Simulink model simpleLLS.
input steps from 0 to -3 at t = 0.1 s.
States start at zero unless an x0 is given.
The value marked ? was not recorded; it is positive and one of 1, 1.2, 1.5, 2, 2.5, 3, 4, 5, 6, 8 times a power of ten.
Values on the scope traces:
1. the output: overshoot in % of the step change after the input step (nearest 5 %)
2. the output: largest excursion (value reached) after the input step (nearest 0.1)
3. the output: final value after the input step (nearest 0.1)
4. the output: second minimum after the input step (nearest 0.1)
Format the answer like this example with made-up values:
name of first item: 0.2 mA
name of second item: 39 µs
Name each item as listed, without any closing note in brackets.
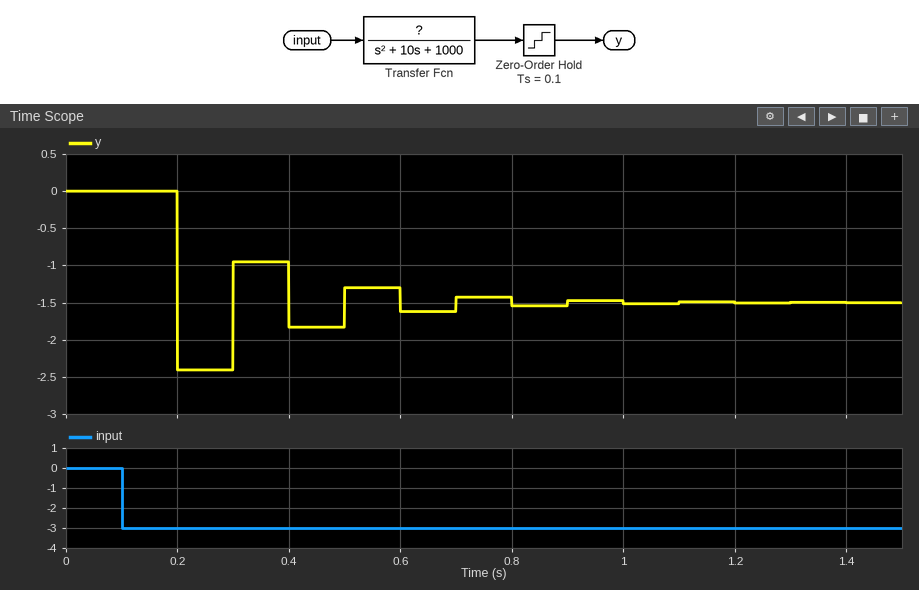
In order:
the output: overshoot in % of the step change after the input step: 60 %
the output: largest excursion (value reached) after the input step: -2.4
the output: final value after the input step: -1.5
the output: second minimum after the input step: -1.8
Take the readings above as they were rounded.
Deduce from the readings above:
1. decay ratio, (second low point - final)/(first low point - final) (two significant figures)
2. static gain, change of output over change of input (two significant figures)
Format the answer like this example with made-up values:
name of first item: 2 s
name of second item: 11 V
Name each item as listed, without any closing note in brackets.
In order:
decay ratio, (second low point - final)/(first low point - final): 0.33
static gain, change of output over change of input: 0.50
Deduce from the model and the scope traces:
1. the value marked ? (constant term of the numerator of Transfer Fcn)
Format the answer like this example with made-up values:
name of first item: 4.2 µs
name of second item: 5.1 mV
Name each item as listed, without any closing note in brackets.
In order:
the value marked ?: 500
